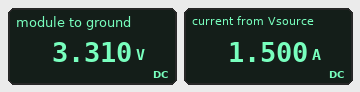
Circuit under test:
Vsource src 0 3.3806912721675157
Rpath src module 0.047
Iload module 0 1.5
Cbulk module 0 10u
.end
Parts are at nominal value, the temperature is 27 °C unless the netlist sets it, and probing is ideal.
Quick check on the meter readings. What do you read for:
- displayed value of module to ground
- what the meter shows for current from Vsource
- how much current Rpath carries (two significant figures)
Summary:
3.310 V
1.500 A
1.5 A
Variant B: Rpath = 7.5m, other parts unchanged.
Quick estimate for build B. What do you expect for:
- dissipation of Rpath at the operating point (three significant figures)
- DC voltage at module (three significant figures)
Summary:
16.9 mW
3.37 V
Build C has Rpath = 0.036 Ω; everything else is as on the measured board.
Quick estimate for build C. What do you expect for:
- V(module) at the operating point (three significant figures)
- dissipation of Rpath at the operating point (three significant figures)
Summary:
3.33 V
81.0 mW
